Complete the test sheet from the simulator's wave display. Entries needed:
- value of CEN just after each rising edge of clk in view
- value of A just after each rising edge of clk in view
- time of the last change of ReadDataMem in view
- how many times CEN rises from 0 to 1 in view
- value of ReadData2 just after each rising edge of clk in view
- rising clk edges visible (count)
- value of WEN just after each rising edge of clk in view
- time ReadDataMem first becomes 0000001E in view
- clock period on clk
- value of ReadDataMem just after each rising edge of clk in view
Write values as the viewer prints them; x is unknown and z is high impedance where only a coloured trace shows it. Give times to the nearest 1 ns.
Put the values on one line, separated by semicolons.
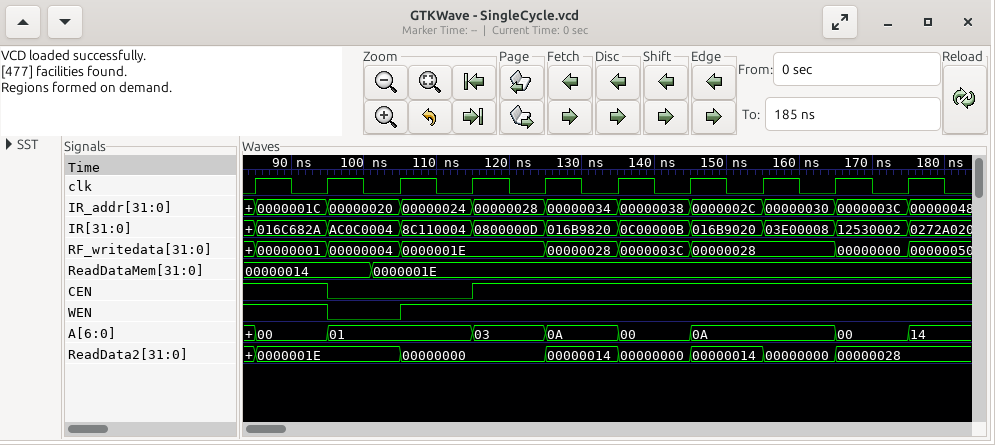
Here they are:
1 0 0 1 1 1 1 1 1 1; 00, 01, 01, 03, 0A, 00, 0A, 0A, 00, 14; 101 ns; 1; 0000001E, 0000001E, 00000000, 00000000, 00000014, 00000000, 00000014, 00000000, 00000028, 00000028; 10; 1 0 1 1 1 1 1 1 1 1; 101 ns; 10 ns; 00000014, 00000014, 0000001E, 0000001E, 0000001E, 0000001E, 0000001E, 0000001E, 0000001E, 0000001E
